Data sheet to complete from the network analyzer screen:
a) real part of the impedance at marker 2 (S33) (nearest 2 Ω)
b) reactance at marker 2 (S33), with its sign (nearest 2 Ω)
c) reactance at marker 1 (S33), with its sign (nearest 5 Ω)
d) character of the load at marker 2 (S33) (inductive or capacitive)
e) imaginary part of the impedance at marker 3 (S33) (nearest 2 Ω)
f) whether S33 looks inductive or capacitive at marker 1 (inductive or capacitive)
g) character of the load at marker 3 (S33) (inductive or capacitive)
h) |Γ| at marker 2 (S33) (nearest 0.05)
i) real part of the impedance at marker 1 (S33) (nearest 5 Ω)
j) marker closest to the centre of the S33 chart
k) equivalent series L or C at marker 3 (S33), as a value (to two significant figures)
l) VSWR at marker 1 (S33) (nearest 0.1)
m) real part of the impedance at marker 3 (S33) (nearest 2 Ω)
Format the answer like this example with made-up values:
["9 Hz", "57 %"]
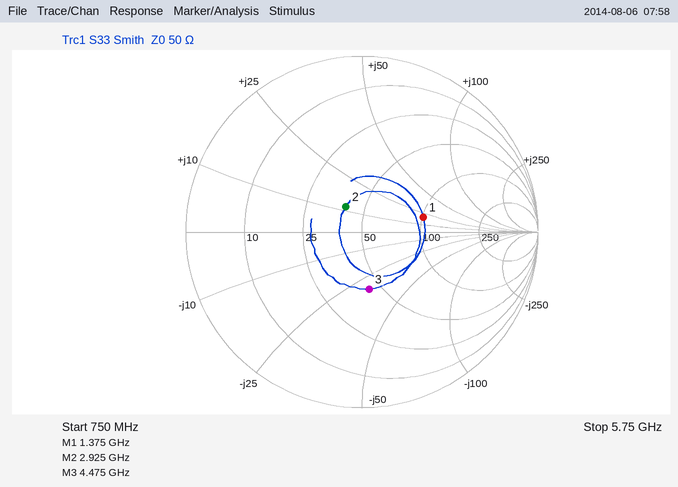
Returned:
["40 Ω", "+12 Ω", "+20 Ω", "inductive", "-32 Ω", "inductive", "capacitive", "0.15", "100 Ω", "marker 2", "1.1 pF", "2.1", "44 Ω"]
